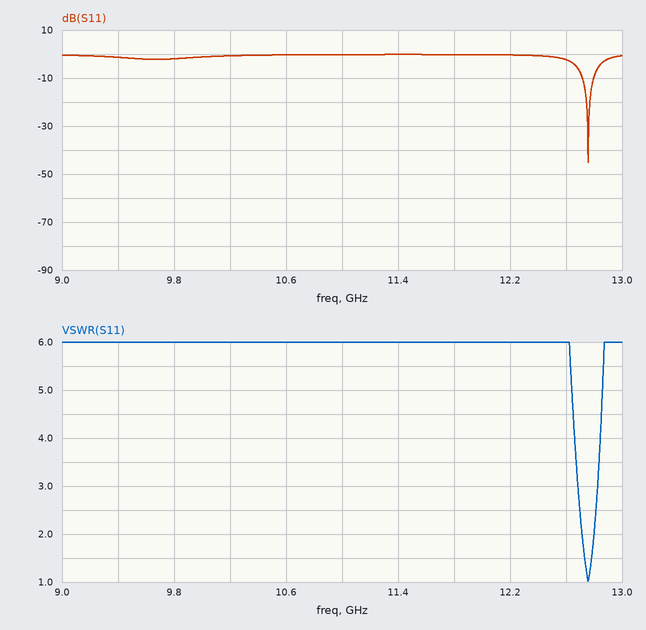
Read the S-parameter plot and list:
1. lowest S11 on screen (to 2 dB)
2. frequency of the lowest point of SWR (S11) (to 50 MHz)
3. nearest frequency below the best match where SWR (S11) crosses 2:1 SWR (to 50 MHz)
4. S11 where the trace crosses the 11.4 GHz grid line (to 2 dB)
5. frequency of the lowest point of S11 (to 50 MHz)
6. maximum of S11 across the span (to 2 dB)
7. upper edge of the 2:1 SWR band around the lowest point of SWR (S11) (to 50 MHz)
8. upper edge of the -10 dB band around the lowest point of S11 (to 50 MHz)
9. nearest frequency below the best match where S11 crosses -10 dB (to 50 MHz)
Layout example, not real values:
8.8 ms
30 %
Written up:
-46 dB
12.75 GHz
12.70 GHz
0 dB
12.75 GHz
0 dB
12.80 GHz
12.80 GHz
12.70 GHz
